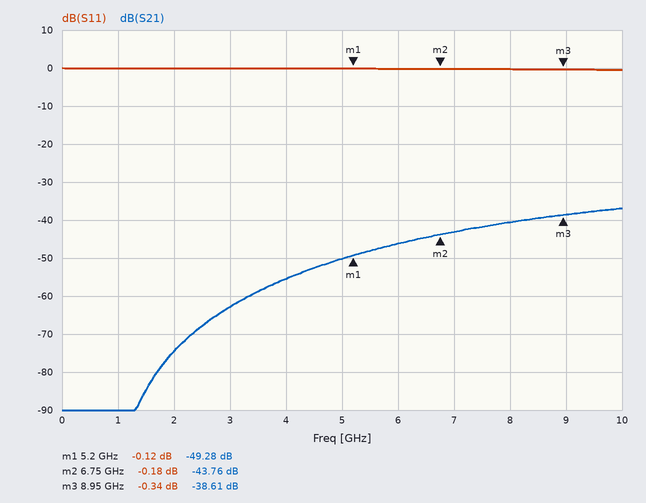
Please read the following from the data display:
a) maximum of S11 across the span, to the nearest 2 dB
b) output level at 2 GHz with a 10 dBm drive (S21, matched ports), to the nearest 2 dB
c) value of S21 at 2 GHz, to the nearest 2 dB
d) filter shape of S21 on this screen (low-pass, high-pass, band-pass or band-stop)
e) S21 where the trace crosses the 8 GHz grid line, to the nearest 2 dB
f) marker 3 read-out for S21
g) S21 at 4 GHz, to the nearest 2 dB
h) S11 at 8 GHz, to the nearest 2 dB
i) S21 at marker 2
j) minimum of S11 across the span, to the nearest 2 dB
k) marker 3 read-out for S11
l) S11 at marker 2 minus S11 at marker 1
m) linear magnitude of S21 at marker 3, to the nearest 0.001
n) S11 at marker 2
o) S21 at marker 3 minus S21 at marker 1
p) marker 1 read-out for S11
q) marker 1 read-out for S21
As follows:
0 dB
-64 dBm
-74 dB
high-pass
-40 dB
-38.61 dB
-56 dB
0 dB
-43.76 dB
0 dB
-0.34 dB
-0.06 dB
0.012
-0.18 dB
10.67 dB
-0.12 dB
-49.28 dB
